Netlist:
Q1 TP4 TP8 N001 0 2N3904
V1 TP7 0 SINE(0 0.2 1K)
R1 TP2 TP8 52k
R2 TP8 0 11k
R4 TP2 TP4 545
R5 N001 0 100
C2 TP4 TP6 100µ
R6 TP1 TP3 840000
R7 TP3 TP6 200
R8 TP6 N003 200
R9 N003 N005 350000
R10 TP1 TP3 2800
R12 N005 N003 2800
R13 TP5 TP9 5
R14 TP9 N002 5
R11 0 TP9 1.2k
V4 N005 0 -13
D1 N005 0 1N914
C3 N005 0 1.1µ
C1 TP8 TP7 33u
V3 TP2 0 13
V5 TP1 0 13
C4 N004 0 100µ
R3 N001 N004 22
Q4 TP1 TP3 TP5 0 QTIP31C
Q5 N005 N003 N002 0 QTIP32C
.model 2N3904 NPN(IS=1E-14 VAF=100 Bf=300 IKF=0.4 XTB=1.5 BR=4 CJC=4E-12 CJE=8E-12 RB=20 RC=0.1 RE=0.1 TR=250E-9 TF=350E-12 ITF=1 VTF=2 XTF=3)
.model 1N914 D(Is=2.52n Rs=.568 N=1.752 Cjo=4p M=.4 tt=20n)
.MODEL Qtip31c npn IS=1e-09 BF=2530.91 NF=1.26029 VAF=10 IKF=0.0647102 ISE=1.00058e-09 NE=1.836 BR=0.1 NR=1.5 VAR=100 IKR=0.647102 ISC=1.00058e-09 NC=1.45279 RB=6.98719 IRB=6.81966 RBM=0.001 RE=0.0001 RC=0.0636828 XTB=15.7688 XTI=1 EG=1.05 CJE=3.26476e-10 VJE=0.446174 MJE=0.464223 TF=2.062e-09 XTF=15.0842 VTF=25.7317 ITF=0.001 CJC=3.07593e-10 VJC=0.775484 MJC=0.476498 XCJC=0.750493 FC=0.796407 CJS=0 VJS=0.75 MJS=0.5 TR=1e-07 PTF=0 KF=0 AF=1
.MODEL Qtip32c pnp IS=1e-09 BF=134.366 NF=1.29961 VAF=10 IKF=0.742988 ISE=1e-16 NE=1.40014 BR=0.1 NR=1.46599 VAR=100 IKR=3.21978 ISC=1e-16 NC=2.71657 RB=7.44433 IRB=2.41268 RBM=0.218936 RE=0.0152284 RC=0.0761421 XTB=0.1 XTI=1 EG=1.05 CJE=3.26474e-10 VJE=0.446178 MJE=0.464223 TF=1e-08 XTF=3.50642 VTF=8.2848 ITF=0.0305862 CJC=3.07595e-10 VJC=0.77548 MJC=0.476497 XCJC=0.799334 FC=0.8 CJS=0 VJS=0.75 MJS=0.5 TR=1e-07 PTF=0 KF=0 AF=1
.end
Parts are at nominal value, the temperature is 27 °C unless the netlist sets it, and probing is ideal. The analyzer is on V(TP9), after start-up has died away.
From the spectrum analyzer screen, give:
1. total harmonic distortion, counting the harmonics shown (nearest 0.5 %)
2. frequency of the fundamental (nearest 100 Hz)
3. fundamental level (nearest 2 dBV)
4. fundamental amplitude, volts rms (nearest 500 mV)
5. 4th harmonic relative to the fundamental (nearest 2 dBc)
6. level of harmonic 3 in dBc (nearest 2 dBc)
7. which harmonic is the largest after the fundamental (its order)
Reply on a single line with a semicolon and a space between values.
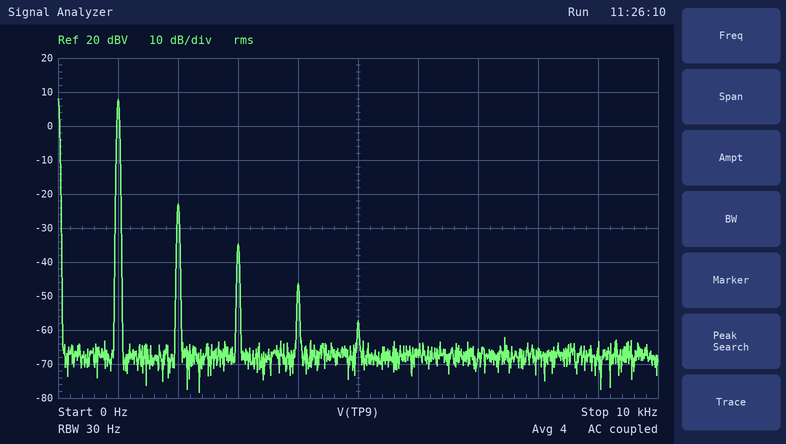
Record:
3.0 %; 1.0 kHz; 8 dBV; 2.5 V; -54 dBc; -42 dBc; 2
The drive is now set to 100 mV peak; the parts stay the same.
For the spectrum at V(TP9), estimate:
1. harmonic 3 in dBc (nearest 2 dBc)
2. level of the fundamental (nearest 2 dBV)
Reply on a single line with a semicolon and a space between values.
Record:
-58 dBc; 2 dBV
